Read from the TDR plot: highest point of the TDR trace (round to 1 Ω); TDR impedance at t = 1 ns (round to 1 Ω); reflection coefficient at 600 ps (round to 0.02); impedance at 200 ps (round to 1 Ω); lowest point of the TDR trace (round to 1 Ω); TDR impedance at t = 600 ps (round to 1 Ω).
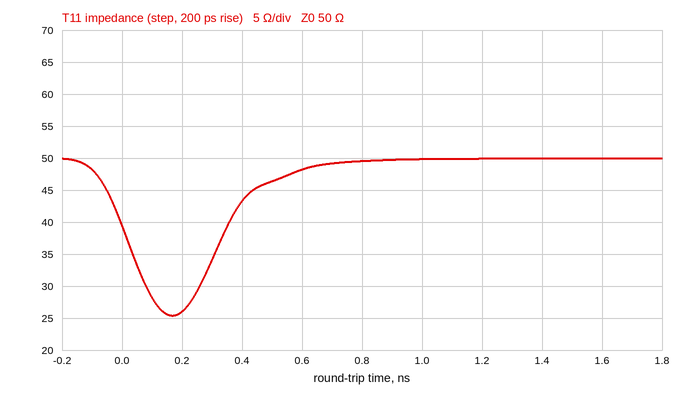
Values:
50 Ω
50 Ω
-0.02
26 Ω
25 Ω
48 Ω
